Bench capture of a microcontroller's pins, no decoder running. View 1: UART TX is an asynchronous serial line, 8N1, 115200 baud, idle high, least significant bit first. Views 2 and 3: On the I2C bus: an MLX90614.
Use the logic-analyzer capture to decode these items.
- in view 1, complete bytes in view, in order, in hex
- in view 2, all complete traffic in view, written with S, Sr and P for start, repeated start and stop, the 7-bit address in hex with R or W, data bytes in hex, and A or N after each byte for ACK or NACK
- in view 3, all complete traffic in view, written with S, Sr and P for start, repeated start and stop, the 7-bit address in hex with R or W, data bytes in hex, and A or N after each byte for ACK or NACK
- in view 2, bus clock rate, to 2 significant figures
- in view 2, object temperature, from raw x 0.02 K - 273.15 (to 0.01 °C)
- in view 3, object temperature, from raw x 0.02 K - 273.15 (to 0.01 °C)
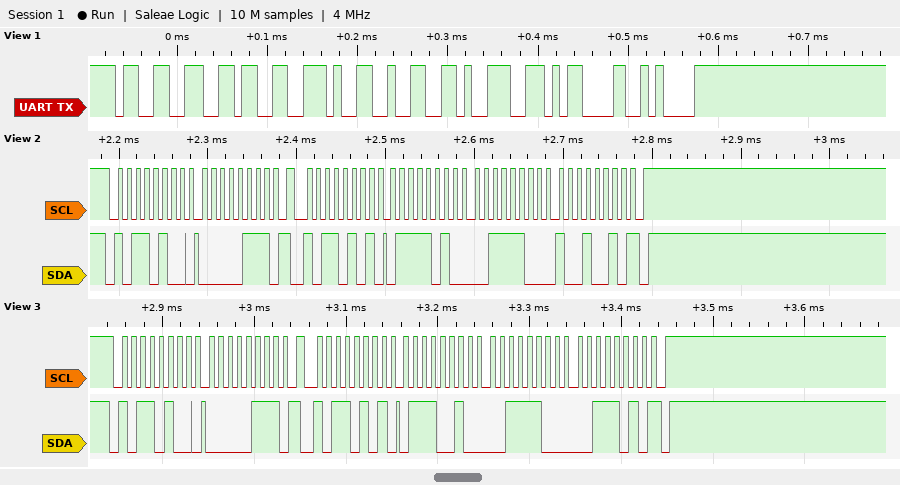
33 36 2E 32 39 0D 0A
S 5AW A 07 A Sr 5AR A 7A A 3C A 92 N P
S 5AW A 07 A Sr 5AR A 72 A 3C A 3A N P
100 kHz
36.49 °C
36.33 °C
